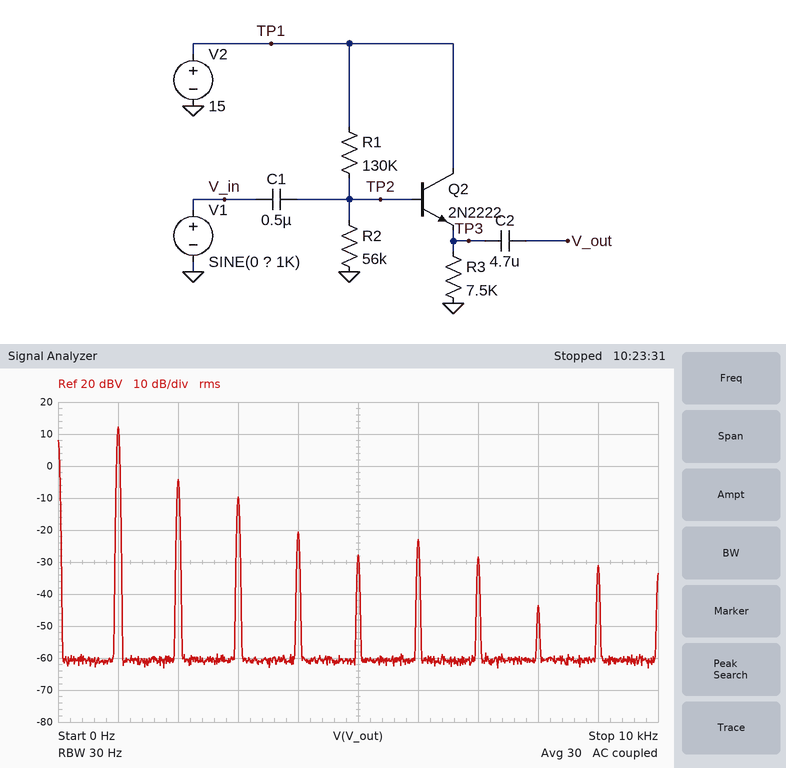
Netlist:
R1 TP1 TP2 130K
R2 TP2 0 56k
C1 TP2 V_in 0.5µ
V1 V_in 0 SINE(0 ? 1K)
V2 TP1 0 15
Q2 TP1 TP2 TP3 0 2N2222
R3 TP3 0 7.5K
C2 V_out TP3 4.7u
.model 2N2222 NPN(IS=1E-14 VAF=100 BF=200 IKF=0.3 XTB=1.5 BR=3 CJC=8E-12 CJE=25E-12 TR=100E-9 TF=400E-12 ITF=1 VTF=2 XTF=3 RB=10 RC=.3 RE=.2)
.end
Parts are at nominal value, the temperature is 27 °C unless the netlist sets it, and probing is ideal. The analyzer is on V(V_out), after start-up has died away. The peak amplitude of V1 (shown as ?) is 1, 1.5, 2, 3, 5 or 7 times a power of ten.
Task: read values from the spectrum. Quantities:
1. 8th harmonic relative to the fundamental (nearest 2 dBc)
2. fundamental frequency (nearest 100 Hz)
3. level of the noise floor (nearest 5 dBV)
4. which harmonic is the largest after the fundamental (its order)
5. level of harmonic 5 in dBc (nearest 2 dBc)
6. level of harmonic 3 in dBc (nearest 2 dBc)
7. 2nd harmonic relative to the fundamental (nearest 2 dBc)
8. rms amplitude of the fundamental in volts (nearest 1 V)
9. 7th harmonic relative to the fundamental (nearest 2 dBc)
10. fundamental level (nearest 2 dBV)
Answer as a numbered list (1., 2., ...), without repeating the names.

1. -56 dBc
2. 1.0 kHz
3. -60 dBV
4. 2
5. -40 dBc
6. -22 dBc
7. -16 dBc
8. 4 V
9. -40 dBc
10. 12 dBV
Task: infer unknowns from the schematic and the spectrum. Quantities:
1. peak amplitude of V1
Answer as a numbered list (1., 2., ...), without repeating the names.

1. 7 V
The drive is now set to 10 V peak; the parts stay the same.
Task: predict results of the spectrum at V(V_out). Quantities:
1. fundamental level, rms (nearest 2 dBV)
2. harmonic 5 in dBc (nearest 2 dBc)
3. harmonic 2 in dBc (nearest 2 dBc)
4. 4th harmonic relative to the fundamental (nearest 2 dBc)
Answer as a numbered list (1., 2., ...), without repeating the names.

1. 14 dBV
2. -30 dBc
3. -12 dBc
4. -44 dBc
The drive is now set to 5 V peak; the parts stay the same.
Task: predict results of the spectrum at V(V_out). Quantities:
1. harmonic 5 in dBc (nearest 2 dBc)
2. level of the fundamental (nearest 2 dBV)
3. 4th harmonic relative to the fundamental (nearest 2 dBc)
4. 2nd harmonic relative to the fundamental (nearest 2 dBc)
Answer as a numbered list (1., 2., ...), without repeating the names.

1. -36 dBc
2. 10 dBV
3. -30 dBc
4. -24 dBc
